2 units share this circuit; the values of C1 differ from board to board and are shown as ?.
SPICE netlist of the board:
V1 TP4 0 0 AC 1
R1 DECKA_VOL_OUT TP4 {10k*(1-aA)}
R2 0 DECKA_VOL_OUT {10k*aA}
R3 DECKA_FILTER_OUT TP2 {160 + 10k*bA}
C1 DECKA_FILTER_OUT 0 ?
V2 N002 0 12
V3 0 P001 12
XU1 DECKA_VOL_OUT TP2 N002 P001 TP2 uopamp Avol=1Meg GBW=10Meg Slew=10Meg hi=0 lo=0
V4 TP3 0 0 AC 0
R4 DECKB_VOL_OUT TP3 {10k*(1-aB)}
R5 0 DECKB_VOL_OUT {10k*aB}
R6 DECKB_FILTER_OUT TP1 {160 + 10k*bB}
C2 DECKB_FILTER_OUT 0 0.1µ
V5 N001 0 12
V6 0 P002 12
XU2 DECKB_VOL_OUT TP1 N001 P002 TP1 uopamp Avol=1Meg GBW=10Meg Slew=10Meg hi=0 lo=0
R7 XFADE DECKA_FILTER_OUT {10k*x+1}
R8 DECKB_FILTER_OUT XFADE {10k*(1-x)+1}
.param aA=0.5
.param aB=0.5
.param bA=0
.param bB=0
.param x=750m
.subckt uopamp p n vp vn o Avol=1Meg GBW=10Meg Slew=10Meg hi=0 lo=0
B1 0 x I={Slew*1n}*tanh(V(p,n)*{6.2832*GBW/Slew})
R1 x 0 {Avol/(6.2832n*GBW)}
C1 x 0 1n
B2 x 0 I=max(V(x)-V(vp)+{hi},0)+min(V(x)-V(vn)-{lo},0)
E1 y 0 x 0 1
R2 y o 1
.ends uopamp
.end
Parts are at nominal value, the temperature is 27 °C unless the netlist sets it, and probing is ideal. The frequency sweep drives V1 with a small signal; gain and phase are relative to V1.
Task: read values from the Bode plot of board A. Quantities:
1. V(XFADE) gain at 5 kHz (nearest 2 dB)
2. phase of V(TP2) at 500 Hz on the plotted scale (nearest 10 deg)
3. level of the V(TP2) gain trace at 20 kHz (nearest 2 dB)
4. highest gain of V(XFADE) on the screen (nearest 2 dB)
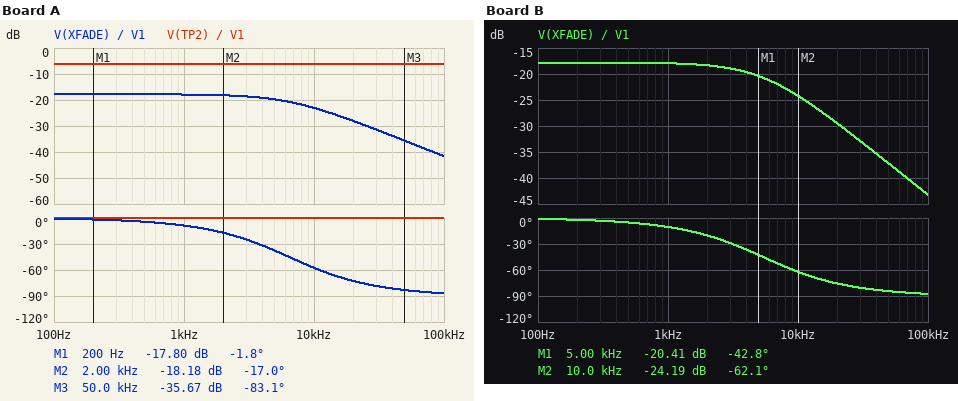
-20 dB
0 deg
-6 dB
-18 dB
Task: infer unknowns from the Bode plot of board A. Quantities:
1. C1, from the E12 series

150 nF
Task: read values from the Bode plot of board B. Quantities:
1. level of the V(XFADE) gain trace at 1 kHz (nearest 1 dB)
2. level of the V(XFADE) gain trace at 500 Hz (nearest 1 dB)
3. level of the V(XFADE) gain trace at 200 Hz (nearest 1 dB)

-18 dB
-18 dB
-18 dB
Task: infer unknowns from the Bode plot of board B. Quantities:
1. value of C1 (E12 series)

180 nF
